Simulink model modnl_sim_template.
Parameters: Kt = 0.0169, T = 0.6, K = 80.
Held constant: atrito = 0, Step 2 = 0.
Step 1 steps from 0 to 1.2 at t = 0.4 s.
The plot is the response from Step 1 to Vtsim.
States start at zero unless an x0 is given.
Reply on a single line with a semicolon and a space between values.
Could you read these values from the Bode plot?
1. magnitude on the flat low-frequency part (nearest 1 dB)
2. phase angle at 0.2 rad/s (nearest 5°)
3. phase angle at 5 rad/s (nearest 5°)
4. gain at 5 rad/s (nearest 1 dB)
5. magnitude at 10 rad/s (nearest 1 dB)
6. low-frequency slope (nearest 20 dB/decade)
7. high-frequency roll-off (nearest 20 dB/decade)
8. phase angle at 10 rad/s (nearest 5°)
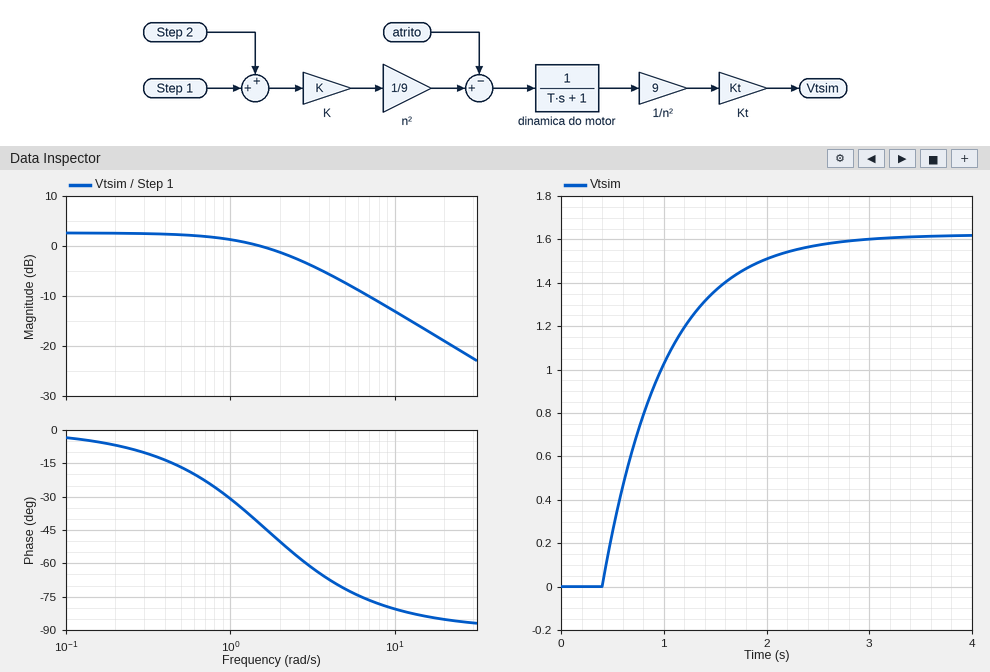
3 dB; -5°; -70°; -7 dB; -13 dB; 0 dB/decade; -20 dB/decade; -80°
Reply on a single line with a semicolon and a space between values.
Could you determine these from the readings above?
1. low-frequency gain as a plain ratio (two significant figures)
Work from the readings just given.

1.4
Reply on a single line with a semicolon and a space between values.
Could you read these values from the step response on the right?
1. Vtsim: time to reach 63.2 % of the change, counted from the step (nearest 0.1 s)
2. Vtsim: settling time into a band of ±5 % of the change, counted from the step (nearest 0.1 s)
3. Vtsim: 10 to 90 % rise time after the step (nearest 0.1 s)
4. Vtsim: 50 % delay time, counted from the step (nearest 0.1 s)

0.6 s; 1.8 s; 1.3 s; 0.4 s
